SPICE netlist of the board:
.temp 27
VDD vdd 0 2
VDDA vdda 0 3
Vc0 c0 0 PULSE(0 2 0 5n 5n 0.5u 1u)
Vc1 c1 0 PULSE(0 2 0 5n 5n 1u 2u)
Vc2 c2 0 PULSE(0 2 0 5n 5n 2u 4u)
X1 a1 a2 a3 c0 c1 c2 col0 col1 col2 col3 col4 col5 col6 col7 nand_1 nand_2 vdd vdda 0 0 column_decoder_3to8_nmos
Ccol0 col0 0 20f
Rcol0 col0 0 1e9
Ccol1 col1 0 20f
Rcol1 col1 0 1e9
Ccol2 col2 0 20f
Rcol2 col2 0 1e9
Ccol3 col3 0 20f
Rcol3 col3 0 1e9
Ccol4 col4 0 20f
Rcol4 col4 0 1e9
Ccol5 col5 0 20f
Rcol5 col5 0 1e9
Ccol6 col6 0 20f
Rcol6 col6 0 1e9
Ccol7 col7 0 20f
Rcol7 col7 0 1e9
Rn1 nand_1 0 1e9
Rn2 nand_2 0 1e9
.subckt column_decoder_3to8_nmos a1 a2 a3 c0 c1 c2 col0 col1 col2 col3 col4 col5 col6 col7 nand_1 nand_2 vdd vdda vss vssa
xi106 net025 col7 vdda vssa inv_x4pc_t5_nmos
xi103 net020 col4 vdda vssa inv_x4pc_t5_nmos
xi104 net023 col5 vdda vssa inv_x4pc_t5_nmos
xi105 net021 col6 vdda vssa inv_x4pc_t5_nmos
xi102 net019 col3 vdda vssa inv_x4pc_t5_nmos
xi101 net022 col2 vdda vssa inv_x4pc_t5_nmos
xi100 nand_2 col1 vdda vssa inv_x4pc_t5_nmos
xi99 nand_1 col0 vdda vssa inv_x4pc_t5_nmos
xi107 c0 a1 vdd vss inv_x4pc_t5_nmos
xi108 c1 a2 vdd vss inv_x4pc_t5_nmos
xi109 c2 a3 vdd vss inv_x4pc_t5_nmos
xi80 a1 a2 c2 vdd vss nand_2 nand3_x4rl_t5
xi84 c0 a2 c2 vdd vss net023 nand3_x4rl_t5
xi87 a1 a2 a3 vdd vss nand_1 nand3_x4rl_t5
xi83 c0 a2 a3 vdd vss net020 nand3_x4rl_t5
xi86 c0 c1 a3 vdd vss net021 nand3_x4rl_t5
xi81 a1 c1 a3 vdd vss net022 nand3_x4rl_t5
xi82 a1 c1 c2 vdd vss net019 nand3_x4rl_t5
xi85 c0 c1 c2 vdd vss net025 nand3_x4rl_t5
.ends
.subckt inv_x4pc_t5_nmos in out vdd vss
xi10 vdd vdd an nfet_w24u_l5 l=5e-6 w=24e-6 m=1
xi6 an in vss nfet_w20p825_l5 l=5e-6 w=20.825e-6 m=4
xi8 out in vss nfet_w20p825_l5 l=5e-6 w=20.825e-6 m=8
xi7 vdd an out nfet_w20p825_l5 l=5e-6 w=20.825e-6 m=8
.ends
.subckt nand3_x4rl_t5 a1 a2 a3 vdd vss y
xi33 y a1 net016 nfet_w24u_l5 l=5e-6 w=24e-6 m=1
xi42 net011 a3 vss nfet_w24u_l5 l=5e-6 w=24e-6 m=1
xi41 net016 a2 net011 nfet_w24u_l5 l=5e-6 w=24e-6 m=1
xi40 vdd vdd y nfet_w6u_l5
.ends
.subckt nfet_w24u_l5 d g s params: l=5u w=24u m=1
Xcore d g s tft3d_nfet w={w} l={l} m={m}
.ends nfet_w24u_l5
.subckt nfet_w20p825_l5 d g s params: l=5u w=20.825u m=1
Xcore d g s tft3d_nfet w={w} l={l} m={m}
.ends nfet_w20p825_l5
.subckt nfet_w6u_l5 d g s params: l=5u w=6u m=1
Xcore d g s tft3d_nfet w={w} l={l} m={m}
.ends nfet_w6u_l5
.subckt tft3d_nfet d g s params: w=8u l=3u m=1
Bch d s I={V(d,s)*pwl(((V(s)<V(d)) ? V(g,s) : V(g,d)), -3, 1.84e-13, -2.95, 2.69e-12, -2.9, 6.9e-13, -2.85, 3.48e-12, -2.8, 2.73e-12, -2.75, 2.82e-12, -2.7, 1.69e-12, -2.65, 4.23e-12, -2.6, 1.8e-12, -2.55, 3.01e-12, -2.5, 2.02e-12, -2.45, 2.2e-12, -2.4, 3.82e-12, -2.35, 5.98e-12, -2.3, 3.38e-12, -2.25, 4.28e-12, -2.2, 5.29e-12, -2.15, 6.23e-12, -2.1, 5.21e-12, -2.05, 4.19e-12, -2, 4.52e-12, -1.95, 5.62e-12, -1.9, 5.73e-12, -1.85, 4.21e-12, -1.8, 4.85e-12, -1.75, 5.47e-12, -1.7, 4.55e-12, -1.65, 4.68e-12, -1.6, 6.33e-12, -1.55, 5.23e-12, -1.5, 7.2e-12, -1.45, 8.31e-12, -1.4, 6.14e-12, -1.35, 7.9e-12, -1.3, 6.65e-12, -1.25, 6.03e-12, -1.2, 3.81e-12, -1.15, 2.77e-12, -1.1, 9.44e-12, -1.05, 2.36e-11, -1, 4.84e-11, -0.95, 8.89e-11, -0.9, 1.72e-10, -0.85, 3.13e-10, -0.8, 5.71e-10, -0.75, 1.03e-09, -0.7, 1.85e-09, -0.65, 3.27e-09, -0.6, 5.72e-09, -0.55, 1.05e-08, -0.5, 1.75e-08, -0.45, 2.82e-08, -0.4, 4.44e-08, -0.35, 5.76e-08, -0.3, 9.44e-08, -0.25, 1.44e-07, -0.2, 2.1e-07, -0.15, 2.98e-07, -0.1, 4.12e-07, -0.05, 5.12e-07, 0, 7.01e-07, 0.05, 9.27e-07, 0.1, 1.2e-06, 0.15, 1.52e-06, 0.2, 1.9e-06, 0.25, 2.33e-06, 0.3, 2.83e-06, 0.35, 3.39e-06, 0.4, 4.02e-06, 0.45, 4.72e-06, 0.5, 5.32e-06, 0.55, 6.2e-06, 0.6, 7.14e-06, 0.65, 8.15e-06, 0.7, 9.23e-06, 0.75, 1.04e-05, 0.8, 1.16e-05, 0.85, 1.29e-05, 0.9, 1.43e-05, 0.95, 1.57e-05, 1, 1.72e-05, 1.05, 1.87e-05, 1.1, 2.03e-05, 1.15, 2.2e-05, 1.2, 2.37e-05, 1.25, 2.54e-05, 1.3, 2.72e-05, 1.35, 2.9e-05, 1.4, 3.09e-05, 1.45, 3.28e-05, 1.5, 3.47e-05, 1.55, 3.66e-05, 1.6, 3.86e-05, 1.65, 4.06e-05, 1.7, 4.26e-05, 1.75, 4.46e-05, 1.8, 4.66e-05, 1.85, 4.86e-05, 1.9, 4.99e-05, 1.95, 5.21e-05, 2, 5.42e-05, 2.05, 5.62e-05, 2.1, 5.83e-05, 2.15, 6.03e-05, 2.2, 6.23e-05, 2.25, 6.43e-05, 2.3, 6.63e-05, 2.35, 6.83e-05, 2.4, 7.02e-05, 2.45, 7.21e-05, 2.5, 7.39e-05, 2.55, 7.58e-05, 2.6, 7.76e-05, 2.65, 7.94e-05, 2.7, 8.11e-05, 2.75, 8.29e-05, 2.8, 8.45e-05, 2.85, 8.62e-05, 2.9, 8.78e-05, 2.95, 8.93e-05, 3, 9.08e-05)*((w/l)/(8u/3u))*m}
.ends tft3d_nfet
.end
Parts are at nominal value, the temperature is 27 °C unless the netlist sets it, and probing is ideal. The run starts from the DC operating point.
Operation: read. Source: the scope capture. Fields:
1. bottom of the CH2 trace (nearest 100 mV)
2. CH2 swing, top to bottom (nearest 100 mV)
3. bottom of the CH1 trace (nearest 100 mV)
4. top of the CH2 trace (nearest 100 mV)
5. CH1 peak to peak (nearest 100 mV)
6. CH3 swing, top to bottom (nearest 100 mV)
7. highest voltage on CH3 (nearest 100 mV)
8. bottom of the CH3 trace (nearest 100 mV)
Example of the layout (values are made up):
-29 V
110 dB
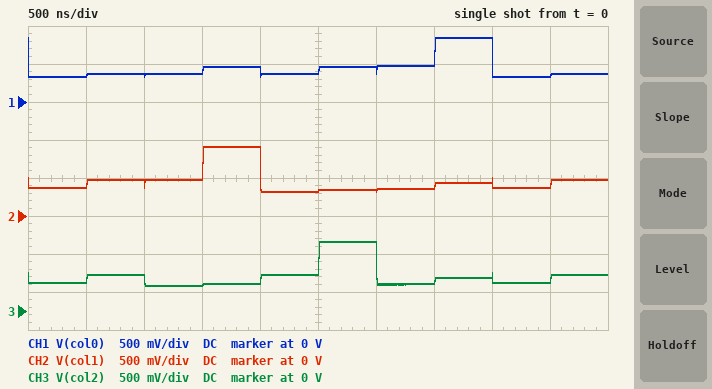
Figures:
300 mV
600 mV
300 mV
900 mV
500 mV
600 mV
900 mV
300 mV
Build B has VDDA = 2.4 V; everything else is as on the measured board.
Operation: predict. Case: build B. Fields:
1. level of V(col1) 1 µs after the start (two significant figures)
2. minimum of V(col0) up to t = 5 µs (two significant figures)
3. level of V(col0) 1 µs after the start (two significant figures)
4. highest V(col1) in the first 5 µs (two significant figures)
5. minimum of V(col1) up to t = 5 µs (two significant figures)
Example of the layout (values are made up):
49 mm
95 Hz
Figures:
280 mV
190 mV
210 mV
590 mV
180 mV
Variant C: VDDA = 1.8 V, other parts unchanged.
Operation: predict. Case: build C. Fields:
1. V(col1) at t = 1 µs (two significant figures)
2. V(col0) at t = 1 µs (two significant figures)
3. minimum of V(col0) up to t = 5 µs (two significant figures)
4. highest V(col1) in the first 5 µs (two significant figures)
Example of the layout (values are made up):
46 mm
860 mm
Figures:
130 mV
96 mV
85 mV
330 mV
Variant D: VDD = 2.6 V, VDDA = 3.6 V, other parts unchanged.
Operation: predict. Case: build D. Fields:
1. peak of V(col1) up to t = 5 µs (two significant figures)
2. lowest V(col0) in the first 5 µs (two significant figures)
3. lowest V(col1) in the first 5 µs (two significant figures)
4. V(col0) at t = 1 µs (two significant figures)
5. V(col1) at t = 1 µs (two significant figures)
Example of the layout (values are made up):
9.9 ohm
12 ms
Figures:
960 mV
350 mV
330 mV
380 mV
480 mV
